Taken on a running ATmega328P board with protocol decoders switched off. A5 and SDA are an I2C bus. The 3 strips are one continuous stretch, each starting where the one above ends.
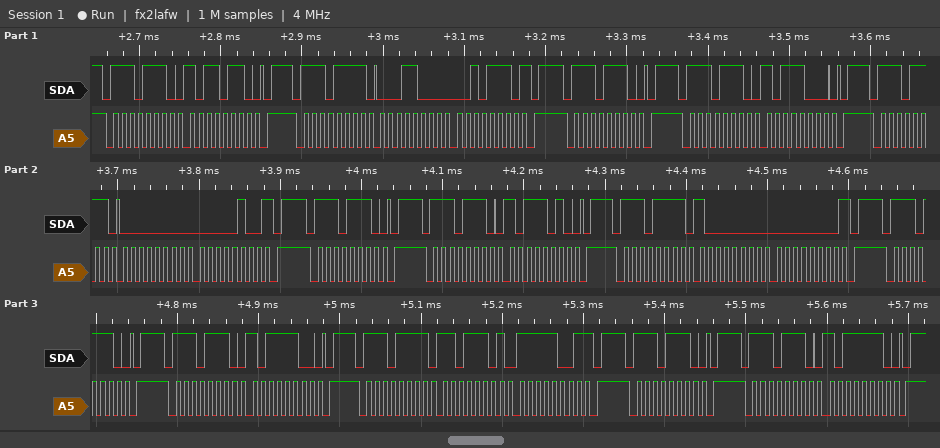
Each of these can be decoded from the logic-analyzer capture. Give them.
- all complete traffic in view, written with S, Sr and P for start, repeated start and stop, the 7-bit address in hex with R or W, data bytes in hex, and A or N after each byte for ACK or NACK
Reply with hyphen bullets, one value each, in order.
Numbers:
- S 77W A B6 A P S 77R A 18 A 2E N P S 77W A P S 77W A B8 A P S 77R A 00 A 04 N P S 77W A P S 77W A BA A P S 77R A 80 A 00 N P S 77W A P S 77W A BC A P S 77R A DD A F9 N P S 77W A P S 77W A BE A P
